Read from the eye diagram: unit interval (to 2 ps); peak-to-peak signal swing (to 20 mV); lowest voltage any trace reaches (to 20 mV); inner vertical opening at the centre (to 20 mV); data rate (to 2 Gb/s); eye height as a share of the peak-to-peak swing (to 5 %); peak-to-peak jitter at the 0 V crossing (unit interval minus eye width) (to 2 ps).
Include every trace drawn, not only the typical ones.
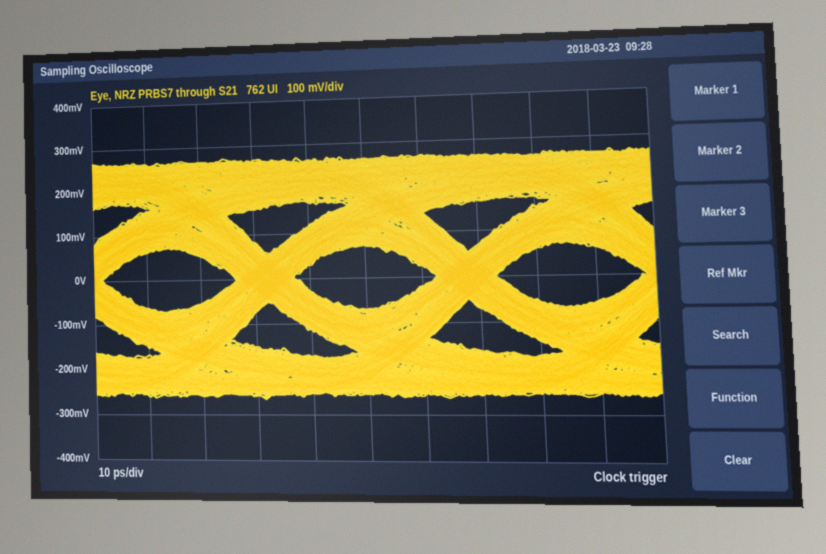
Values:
36 ps
540 mV
-260 mV
140 mV
28 Gb/s
25 %
10 ps
